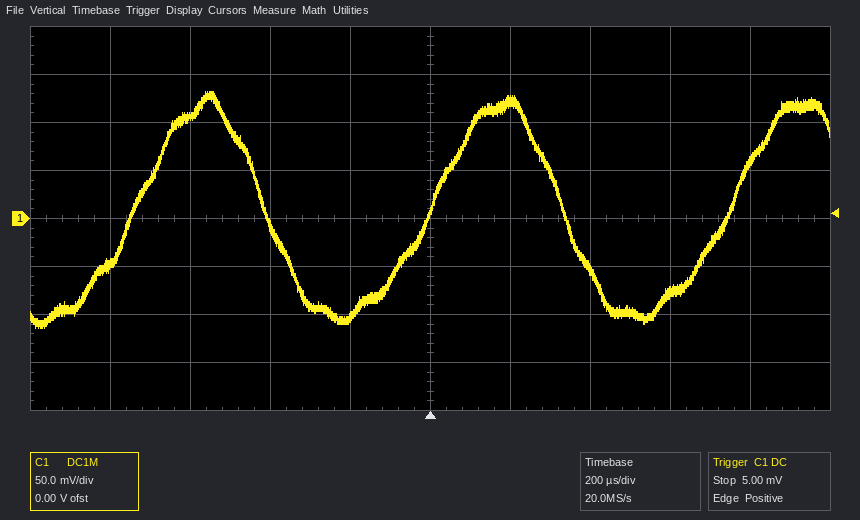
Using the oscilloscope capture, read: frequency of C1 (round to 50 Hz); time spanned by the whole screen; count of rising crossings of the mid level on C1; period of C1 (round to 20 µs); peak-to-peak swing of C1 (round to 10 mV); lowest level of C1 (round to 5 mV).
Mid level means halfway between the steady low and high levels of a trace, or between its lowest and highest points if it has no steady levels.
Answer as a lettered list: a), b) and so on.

a) 1.35 kHz
b) 2 ms
c) 3
d) 740 µs
e) 250 mV
f) -115 mV
